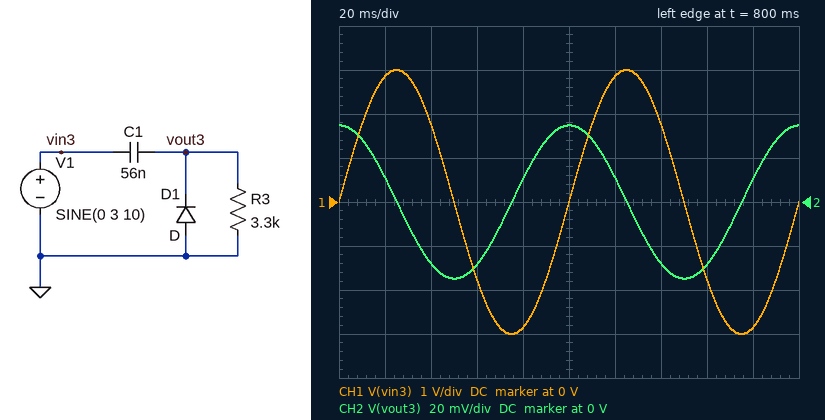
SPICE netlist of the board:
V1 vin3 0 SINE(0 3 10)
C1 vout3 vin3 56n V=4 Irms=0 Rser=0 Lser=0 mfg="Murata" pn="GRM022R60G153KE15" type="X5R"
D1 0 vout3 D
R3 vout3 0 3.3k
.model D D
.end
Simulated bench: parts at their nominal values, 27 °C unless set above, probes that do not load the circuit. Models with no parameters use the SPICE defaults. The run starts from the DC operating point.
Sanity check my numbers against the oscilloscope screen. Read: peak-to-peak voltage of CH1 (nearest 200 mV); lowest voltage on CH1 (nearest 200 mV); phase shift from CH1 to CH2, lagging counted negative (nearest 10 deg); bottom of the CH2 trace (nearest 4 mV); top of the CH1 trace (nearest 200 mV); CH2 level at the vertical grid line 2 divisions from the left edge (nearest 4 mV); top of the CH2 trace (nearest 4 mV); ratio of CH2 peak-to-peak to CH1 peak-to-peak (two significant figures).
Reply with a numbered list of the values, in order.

1. 6.0 V
2. -3.0 V
3. 90 deg
4. -36 mV
5. 3.0 V
6. -28 mV
7. 36 mV
8. 0.012
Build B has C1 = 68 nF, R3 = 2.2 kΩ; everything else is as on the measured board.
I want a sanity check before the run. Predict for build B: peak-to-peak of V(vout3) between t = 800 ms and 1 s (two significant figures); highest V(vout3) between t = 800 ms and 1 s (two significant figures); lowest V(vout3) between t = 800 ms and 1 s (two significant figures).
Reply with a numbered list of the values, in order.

1. 56 mV
2. 28 mV
3. -28 mV
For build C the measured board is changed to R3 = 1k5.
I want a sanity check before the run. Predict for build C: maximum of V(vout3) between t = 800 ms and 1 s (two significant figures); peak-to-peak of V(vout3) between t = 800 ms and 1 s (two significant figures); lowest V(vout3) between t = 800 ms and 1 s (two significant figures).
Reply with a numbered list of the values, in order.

1. 16 mV
2. 32 mV
3. -16 mV
